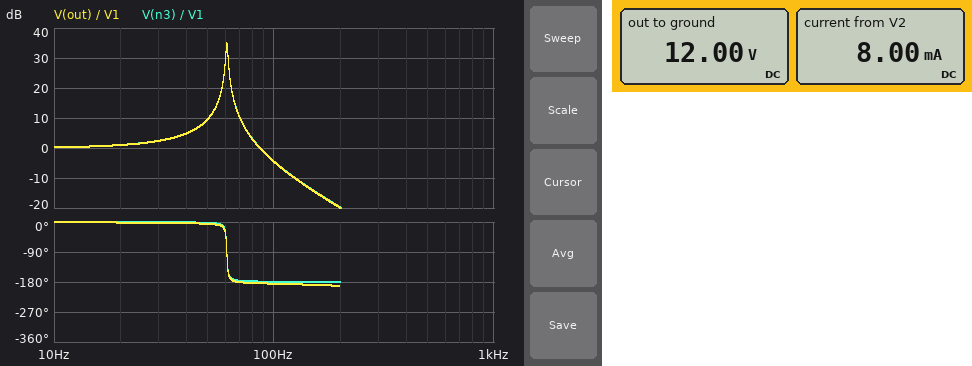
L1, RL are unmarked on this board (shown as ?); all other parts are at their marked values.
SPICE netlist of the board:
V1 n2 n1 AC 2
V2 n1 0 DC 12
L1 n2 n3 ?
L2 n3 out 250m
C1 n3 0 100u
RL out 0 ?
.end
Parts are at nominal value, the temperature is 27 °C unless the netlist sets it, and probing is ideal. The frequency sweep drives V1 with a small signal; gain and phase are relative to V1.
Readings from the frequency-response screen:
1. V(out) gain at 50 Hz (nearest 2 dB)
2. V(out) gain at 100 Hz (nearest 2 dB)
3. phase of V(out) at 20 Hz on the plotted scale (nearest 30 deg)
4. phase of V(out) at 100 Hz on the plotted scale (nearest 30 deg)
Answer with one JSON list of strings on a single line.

["10 dB", "-4 dB", "0 deg", "-180 deg"]
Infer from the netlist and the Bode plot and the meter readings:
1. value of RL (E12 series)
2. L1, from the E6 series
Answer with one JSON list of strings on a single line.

["1.5 kΩ", "68 mH"]
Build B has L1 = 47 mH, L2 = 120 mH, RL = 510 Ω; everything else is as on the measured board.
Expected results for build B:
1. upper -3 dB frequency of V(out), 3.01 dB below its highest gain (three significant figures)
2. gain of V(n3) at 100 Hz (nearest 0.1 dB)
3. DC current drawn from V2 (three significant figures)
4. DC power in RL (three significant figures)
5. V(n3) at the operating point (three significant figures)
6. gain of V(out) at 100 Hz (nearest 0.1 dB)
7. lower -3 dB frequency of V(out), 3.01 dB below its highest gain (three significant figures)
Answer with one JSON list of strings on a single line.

["75.1 Hz", "1.4 dB", "23.5 mA", "282 mW", "12.0 V", "1.3 dB", "72.0 Hz"]
